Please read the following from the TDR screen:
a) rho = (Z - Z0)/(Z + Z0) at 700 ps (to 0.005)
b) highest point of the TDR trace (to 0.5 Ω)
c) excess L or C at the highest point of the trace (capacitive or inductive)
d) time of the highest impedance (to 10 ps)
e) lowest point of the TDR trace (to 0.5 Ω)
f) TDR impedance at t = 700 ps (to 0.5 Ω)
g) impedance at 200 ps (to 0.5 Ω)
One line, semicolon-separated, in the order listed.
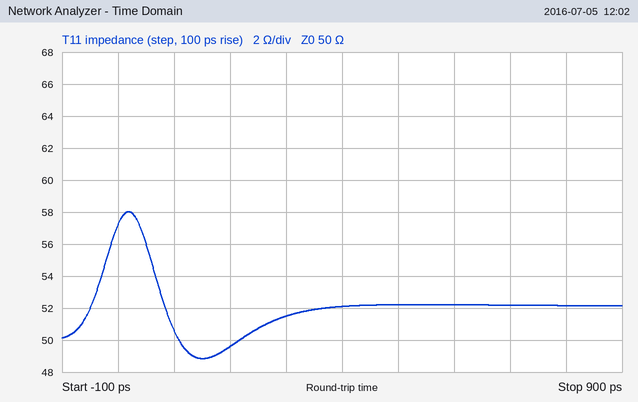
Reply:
+0.020; 58.0 Ω; inductive; 20 ps; 49.0 Ω; 52.0 Ω; 49.5 Ω
